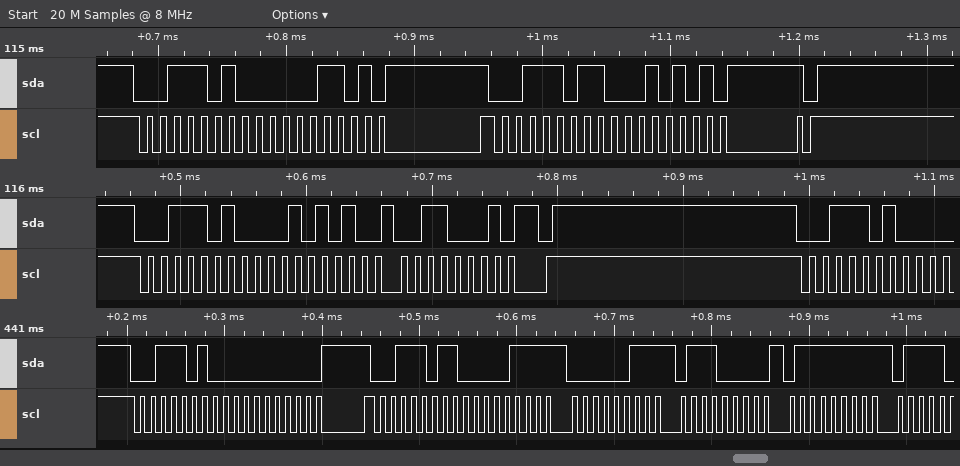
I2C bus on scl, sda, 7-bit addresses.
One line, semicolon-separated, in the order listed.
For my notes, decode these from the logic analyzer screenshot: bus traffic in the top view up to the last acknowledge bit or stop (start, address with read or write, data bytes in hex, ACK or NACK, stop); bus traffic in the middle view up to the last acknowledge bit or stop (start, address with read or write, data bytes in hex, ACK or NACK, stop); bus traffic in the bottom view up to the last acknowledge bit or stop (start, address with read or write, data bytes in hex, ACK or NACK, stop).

start, address 1D write ACK, 0D ACK, repeated start, address 1D read ACK, 2A NACK, stop; start, address 1D write ACK, 2A ACK, 31 ACK, stop, start, address 1D write ACK; start, address 1D write ACK, 00 ACK, repeated start, address 1D read ACK, 0F ACK, 07 ACK, E0 ACK, FF ACK
